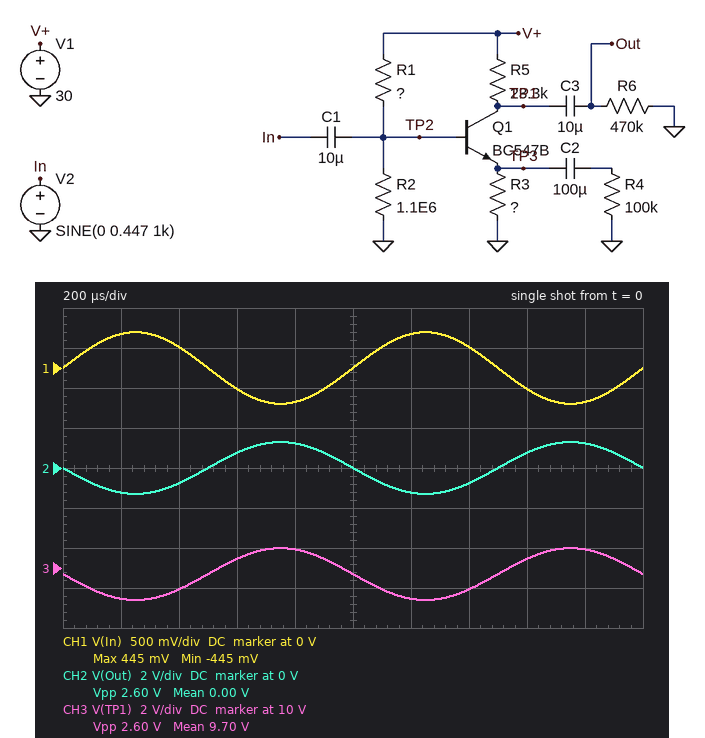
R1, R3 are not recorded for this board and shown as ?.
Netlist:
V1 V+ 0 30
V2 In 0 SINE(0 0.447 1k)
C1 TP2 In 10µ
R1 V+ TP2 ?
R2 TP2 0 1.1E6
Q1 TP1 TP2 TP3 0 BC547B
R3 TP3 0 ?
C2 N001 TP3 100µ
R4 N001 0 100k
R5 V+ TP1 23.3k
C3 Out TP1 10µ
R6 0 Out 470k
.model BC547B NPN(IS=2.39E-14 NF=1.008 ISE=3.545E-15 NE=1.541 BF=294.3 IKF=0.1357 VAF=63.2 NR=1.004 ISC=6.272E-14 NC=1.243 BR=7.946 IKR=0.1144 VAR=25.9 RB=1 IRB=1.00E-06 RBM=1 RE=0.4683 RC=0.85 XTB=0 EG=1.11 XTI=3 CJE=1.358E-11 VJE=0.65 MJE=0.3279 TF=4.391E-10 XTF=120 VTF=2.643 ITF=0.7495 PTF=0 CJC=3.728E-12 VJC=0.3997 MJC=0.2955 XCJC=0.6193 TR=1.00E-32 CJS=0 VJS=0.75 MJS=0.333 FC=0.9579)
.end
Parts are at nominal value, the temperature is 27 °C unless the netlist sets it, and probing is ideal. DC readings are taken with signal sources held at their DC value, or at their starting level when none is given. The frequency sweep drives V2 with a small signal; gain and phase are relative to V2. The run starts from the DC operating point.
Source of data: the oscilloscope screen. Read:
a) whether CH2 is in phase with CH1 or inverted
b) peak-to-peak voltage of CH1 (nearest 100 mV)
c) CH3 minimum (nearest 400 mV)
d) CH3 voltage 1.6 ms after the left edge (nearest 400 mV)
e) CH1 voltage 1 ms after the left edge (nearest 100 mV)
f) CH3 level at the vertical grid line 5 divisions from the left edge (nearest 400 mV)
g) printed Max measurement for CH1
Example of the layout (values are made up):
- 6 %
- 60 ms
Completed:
- inverted
- 900 mV
- 8.4 V
- 10.4 V
- 0 V
- 9.6 V
- 445 mV
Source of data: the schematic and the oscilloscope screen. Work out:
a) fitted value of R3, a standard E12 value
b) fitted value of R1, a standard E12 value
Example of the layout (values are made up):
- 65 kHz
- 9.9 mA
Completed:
- 8.2 kΩ
- 2.2 MΩ
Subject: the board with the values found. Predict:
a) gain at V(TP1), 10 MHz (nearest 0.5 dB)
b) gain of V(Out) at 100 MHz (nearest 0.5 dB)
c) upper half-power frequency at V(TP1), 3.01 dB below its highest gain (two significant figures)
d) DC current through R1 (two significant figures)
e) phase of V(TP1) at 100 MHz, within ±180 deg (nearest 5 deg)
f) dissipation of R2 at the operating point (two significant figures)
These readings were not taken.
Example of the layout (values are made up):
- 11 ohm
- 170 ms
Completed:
- 2.5 dB
- 0.5 dB
- 3.8 MHz
- 10 µA
- 5 deg
- 55 µW
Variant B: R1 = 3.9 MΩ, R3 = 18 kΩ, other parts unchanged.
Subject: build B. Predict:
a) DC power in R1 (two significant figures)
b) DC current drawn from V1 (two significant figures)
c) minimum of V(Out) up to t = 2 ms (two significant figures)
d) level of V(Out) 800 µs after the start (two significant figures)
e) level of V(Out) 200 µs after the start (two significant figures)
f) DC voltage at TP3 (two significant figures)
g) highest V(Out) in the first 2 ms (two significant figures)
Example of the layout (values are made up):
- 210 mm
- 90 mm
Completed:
- 150 µW
- 300 µA
- -640 mV
- 610 mV
- -610 mV
- 5.3 V
- 640 mV
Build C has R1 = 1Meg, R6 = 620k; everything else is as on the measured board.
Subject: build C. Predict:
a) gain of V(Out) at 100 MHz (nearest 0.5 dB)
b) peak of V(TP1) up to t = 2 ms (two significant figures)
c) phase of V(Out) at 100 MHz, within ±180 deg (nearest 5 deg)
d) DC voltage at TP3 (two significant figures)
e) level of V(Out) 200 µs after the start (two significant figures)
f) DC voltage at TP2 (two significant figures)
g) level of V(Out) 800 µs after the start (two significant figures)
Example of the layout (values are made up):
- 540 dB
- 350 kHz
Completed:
- 0 dB
- 9.0 V
- 0 deg
- 7.9 V
- 370 mV
- 8.5 V
- 1.0 V
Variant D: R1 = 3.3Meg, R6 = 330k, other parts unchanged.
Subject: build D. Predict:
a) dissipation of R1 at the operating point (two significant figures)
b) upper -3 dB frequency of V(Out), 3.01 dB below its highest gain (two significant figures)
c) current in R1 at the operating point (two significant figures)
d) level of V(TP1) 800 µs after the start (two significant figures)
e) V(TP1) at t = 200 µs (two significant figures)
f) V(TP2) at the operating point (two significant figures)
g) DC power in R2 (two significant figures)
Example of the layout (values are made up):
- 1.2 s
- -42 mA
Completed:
- 180 µW
- 6.1 MHz
- 7.3 µA
- 16 V
- 14 V
- 5.9 V
- 31 µW
